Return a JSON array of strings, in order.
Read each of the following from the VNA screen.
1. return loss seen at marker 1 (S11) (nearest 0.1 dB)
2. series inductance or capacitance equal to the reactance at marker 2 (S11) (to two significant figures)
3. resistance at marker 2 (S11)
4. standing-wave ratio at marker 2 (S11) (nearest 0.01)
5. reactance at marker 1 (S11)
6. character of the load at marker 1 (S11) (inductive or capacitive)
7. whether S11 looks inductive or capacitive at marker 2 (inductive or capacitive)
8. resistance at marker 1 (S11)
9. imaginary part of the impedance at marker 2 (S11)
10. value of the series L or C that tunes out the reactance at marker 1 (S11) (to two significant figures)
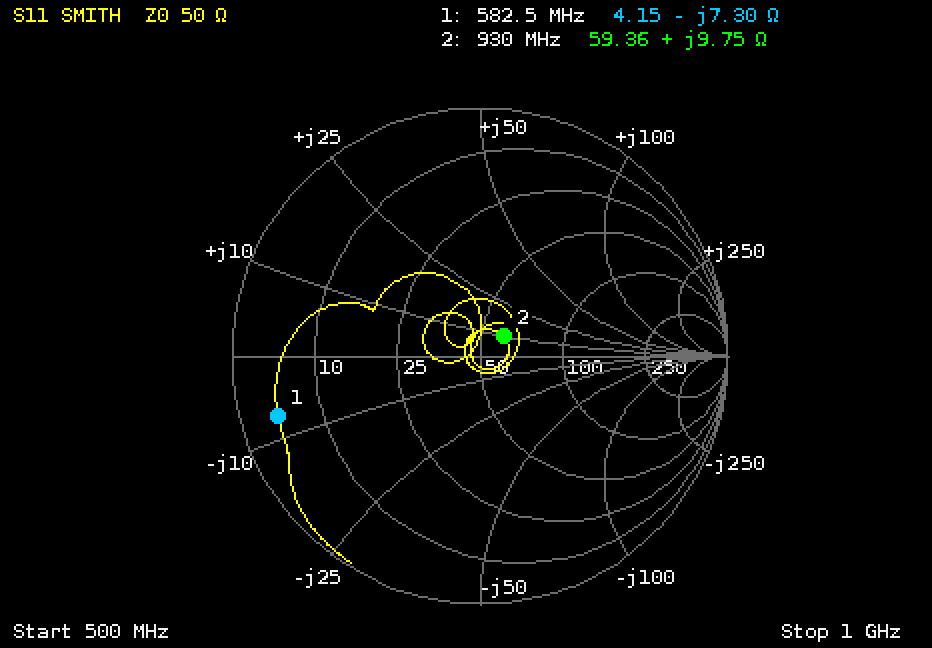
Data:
["1.4 dB", "1.7 nH", "59.36 Ω", "1.28", "-7.30 Ω", "capacitive", "inductive", "4.15 Ω", "+9.75 Ω", "2.0 nH"]
